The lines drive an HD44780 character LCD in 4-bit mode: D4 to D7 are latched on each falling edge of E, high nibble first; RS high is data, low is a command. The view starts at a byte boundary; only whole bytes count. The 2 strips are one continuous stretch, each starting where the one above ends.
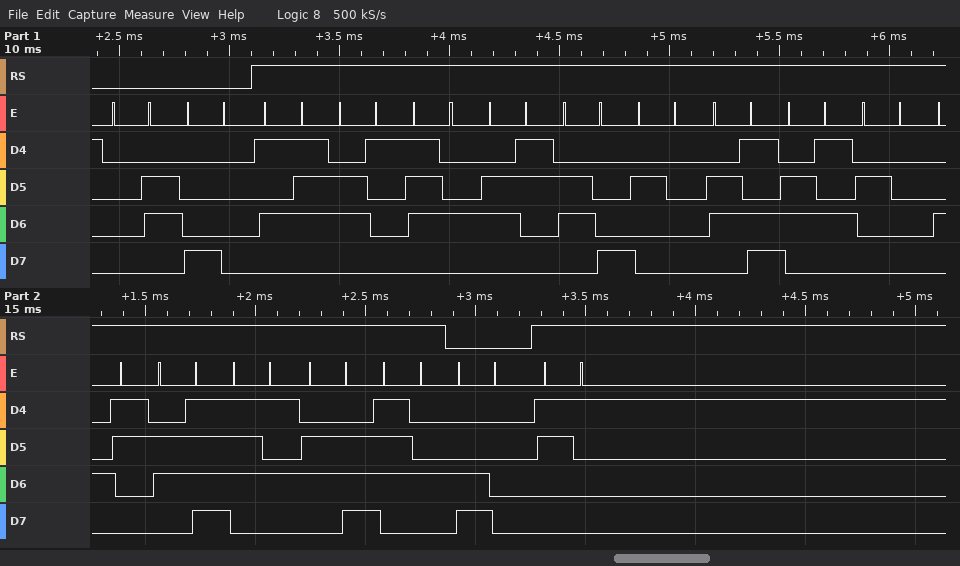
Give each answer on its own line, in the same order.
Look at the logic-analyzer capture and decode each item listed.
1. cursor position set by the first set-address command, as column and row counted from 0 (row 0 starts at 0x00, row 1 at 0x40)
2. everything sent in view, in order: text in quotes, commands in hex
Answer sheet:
column 0, row 0
0x06 0x80 "Watch me Count" 0xC0 "1"
